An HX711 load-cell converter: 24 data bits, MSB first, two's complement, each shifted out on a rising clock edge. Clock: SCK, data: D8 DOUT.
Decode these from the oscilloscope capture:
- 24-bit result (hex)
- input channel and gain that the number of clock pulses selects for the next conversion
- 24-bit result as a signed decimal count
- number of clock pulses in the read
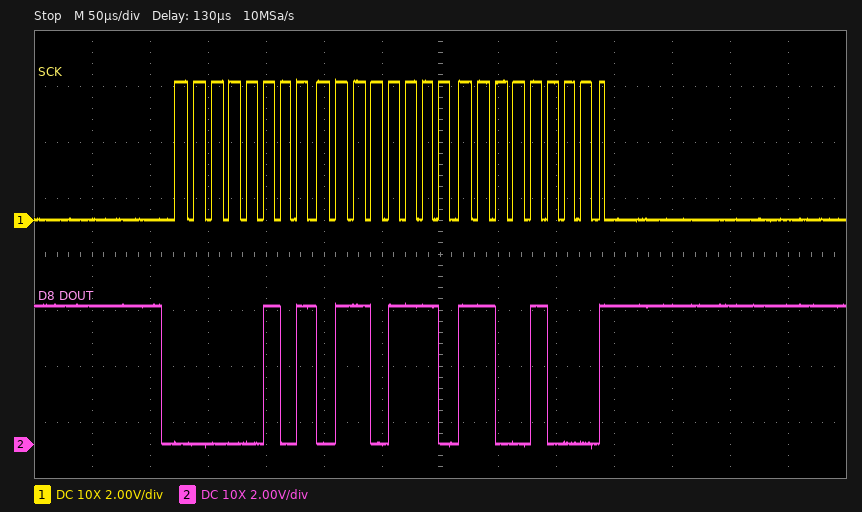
0x056EC8
channel A, gain 128
356040
25
